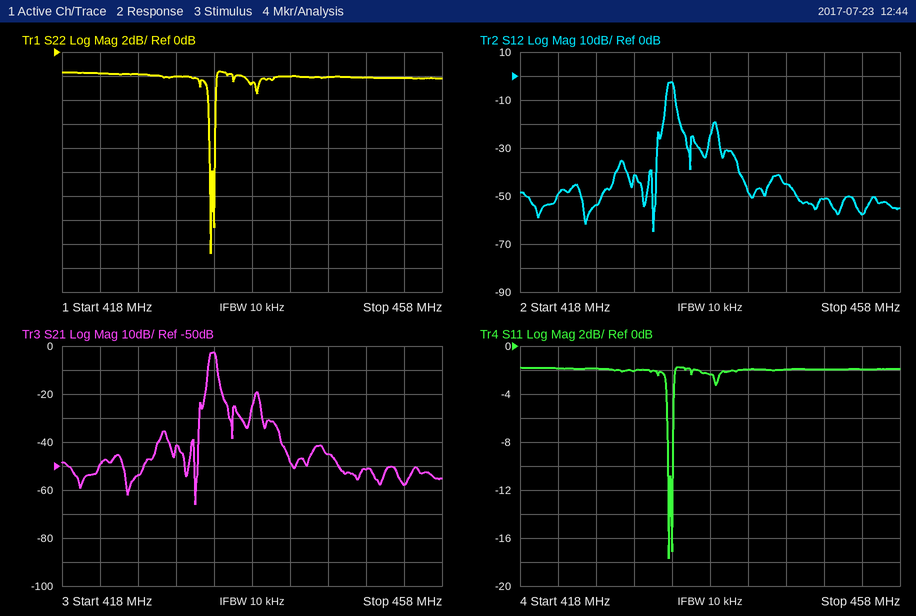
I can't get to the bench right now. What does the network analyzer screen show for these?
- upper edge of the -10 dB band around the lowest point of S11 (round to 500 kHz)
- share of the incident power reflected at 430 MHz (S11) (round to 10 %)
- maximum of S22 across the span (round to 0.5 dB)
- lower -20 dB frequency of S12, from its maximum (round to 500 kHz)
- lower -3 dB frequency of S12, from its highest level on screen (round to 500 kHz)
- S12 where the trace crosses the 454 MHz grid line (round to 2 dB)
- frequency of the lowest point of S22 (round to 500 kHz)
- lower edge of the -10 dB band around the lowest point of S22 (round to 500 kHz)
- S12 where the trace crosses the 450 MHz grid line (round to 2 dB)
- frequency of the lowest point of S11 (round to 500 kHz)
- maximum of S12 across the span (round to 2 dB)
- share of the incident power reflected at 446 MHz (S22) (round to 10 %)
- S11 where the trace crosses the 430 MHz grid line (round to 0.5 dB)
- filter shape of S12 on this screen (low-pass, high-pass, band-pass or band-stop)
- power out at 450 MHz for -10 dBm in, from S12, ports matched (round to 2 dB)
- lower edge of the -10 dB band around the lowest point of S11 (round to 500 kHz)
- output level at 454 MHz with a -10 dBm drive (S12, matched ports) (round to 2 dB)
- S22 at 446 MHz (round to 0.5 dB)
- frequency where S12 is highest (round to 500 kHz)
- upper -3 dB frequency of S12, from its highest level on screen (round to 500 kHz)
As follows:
434.0 MHz
60 %
-1.5 dB
433.0 MHz
433.5 MHz
-58 dB
433.5 MHz
433.5 MHz
-52 dB
433.5 MHz
-2 dB
60 %
-2.0 dB
band-pass
-62 dBm
433.5 MHz
-68 dBm
-2.0 dB
434.0 MHz
434.0 MHz
